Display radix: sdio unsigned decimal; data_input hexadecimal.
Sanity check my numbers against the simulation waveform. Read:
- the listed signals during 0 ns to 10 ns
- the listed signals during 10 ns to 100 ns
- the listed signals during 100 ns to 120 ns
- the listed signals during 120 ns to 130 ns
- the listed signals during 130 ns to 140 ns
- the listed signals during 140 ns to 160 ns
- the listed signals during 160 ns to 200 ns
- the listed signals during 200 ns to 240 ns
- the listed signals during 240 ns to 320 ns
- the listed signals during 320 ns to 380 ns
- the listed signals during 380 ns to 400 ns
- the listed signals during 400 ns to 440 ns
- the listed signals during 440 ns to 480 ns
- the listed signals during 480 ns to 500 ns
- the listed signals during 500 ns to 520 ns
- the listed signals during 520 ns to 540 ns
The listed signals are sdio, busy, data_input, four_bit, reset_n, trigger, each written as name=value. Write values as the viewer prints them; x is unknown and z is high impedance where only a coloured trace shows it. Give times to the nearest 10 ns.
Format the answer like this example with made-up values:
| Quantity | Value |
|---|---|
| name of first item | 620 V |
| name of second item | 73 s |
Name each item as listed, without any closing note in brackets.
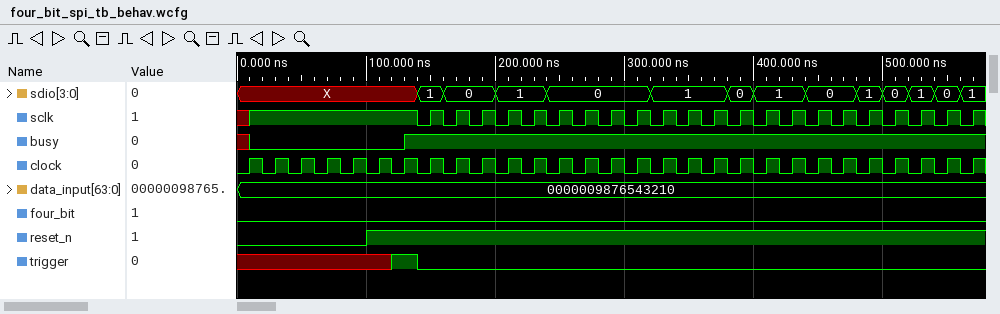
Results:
| Quantity | Value |
|---|---|
| the listed signals during 0 ns to 10 ns | sdio=X, busy=x, data_input=0000009876543210, four_bit=0, reset_n=0, trigger=x |
| the listed signals during 10 ns to 100 ns | sdio=X, busy=0, data_input=0000009876543210, four_bit=0, reset_n=0, trigger=x |
| the listed signals during 100 ns to 120 ns | sdio=X, busy=0, data_input=0000009876543210, four_bit=0, reset_n=1, trigger=x |
| the listed signals during 120 ns to 130 ns | sdio=X, busy=0, data_input=0000009876543210, four_bit=0, reset_n=1, trigger=1 |
| the listed signals during 130 ns to 140 ns | sdio=X, busy=1, data_input=0000009876543210, four_bit=0, reset_n=1, trigger=1 |
| the listed signals during 140 ns to 160 ns | sdio=1, busy=1, data_input=0000009876543210, four_bit=0, reset_n=1, trigger=0 |
| the listed signals during 160 ns to 200 ns | sdio=0, busy=1, data_input=0000009876543210, four_bit=0, reset_n=1, trigger=0 |
| the listed signals during 200 ns to 240 ns | sdio=1, busy=1, data_input=0000009876543210, four_bit=0, reset_n=1, trigger=0 |
| the listed signals during 240 ns to 320 ns | sdio=0, busy=1, data_input=0000009876543210, four_bit=0, reset_n=1, trigger=0 |
| the listed signals during 320 ns to 380 ns | sdio=1, busy=1, data_input=0000009876543210, four_bit=0, reset_n=1, trigger=0 |
| the listed signals during 380 ns to 400 ns | sdio=0, busy=1, data_input=0000009876543210, four_bit=0, reset_n=1, trigger=0 |
| the listed signals during 400 ns to 440 ns | sdio=1, busy=1, data_input=0000009876543210, four_bit=0, reset_n=1, trigger=0 |
| the listed signals during 440 ns to 480 ns | sdio=0, busy=1, data_input=0000009876543210, four_bit=0, reset_n=1, trigger=0 |
| the listed signals during 480 ns to 500 ns | sdio=1, busy=1, data_input=0000009876543210, four_bit=0, reset_n=1, trigger=0 |
| the listed signals during 500 ns to 520 ns | sdio=0, busy=1, data_input=0000009876543210, four_bit=0, reset_n=1, trigger=0 |
| the listed signals during 520 ns to 540 ns | sdio=1, busy=1, data_input=0000009876543210, four_bit=0, reset_n=1, trigger=0 |
